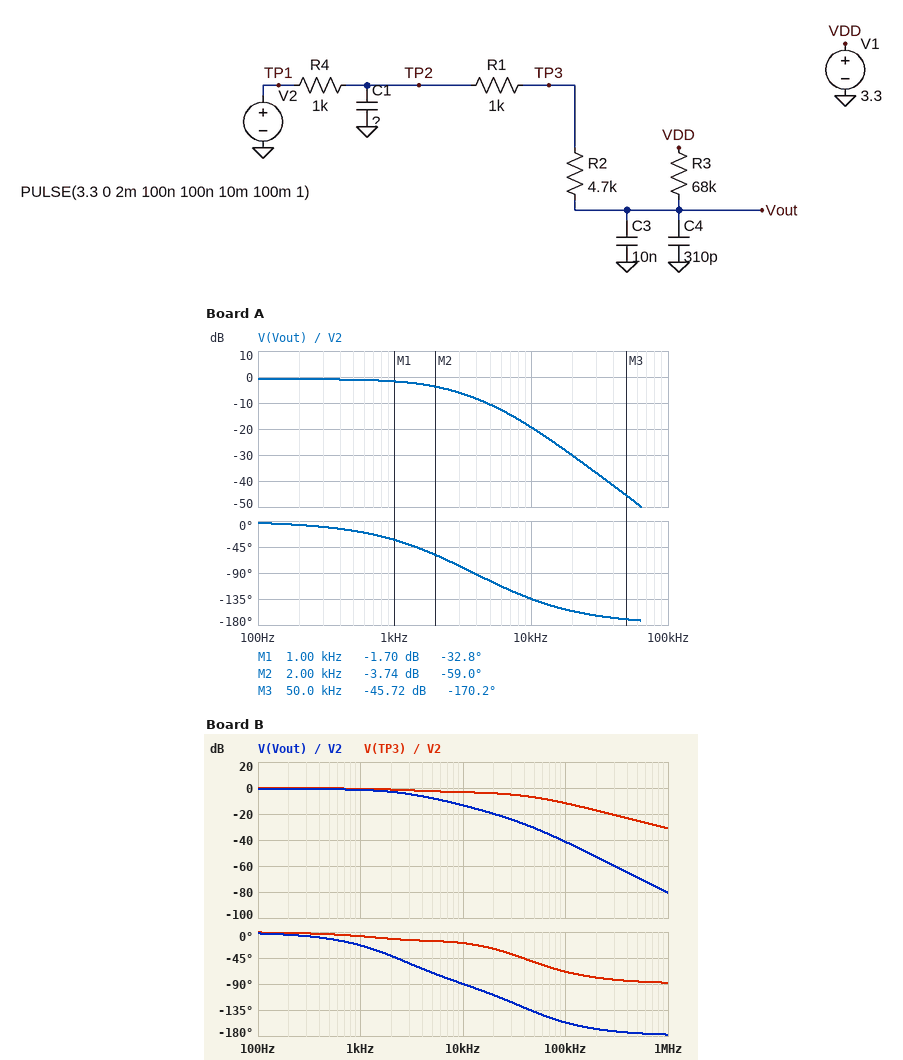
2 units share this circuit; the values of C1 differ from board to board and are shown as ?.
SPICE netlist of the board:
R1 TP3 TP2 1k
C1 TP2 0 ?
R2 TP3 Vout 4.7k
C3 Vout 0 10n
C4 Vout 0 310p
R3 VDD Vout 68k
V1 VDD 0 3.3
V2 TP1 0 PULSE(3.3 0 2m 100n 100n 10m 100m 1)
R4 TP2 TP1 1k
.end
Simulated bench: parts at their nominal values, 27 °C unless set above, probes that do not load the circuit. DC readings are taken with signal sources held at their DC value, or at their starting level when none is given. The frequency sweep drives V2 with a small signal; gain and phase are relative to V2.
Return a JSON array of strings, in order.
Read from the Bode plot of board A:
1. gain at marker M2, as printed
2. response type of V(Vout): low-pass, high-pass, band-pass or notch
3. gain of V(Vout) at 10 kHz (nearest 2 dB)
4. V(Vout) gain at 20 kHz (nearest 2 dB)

["-3.74 dB", "low-pass", "-20 dB", "-30 dB"]
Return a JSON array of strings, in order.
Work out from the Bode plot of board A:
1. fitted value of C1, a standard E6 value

["33 nF"]
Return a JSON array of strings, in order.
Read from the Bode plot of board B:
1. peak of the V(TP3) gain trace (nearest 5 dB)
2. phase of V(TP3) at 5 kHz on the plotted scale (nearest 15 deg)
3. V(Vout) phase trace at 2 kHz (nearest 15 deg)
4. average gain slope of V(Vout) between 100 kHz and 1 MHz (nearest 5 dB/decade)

["0 dB", "-15 deg", "-45 deg", "-40 dB/decade"]
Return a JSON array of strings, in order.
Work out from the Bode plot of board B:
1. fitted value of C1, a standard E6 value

["4.7 nF"]
